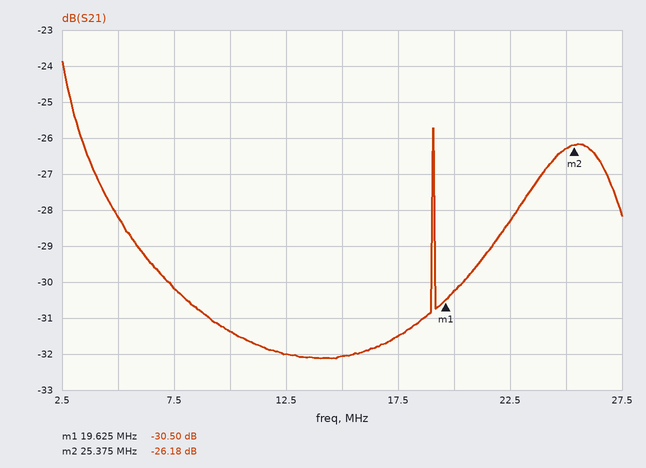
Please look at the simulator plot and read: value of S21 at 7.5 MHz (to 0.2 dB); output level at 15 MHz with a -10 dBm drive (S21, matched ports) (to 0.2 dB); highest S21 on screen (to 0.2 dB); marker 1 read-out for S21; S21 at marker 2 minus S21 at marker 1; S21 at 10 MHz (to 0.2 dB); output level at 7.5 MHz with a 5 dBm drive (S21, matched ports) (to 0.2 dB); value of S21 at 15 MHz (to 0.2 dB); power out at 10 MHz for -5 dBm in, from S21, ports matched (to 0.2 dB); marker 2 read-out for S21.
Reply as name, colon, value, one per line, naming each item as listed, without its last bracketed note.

value of S21 at 7.5 MHz: -30.2 dB
output level at 15 MHz with a -10 dBm drive (S21, matched ports): -42.0 dBm
highest S21 on screen: -23.8 dB
marker 1 read-out for S21: -30.50 dB
S21 at marker 2 minus S21 at marker 1: 4.32 dB
S21 at 10 MHz: -31.4 dB
output level at 7.5 MHz with a 5 dBm drive (S21, matched ports): -25.2 dBm
value of S21 at 15 MHz: -32.0 dB
power out at 10 MHz for -5 dBm in, from S21, ports matched: -36.4 dBm
marker 2 read-out for S21: -26.18 dB
